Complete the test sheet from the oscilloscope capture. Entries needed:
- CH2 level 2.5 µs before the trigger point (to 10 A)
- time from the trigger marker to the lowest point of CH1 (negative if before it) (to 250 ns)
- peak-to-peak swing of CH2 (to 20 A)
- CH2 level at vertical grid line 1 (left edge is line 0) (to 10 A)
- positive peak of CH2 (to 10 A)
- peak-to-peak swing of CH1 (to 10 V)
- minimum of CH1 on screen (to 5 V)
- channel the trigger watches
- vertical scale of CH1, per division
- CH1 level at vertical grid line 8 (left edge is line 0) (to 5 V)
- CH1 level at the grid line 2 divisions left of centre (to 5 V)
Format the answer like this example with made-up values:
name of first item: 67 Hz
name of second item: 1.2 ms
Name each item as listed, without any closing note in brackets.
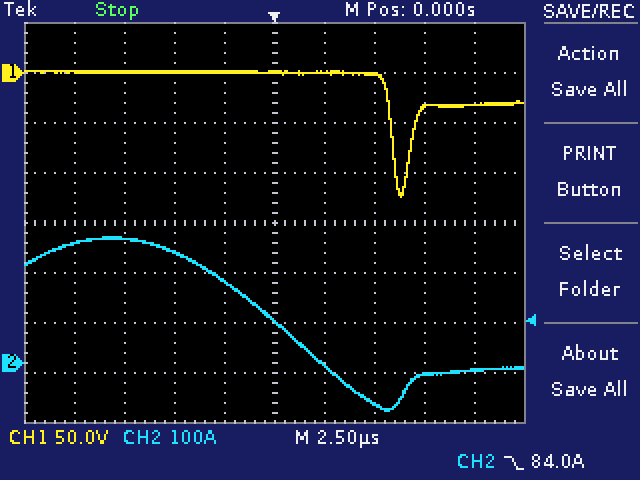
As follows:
CH2 level 2.5 µs before the trigger point: 160 A
time from the trigger marker to the lowest point of CH1 (negative if before it): +6.25 µs
peak-to-peak swing of CH2: 340 A
CH2 level at vertical grid line 1 (left edge is line 0): 240 A
positive peak of CH2: 250 A
peak-to-peak swing of CH1: 130 V
minimum of CH1 on screen: -125 V
channel the trigger watches: CH2
vertical scale of CH1, per division: 50 V
CH1 level at vertical grid line 8 (left edge is line 0): -35 V
CH1 level at the grid line 2 divisions left of centre: 0 V
